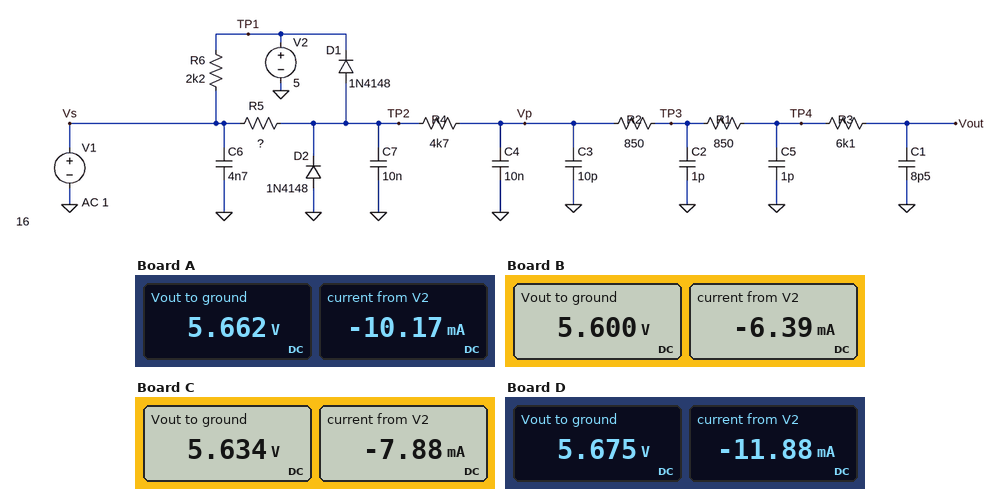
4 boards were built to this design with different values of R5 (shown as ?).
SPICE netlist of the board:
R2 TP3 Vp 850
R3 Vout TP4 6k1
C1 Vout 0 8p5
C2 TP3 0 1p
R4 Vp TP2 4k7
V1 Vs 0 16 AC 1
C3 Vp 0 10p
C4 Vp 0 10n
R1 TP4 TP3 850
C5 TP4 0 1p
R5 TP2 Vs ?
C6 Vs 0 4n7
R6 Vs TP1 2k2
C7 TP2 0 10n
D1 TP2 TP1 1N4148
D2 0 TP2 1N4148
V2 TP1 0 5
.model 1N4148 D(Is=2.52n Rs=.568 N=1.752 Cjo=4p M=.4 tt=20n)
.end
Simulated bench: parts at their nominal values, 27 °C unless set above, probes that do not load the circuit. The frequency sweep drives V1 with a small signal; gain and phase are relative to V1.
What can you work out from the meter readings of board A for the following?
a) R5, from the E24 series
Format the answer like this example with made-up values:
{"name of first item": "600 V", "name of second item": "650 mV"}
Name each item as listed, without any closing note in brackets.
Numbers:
{"R5, from the E24 series": "2 kΩ"}
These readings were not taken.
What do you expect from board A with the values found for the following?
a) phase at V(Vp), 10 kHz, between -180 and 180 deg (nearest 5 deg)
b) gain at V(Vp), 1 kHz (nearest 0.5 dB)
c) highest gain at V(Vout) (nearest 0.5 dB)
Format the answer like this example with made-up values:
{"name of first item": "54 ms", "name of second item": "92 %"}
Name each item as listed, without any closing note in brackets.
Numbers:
{"phase at V(Vp), 10 kHz, between -180 and 180 deg": "-70 deg", "gain at V(Vp), 1 kHz": "-47.0 dB", "highest gain at V(Vout)": "-46.5 dB"}
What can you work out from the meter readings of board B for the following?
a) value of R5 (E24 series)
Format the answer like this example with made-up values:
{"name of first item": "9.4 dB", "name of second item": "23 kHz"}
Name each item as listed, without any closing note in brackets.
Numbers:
{"value of R5": "7.5 kΩ"}
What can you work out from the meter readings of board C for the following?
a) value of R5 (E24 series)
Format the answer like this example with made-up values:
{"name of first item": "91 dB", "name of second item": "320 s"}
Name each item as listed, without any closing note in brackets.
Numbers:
{"value of R5": "3.6 kΩ"}
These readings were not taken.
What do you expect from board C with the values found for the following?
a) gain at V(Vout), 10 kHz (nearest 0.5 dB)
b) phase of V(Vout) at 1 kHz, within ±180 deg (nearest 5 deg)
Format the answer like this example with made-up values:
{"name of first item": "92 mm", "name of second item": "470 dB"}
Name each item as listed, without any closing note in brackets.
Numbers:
{"gain at V(Vout), 10 kHz": "-57.0 dB", "phase of V(Vout) at 1 kHz, within ±180 deg": "-15 deg"}
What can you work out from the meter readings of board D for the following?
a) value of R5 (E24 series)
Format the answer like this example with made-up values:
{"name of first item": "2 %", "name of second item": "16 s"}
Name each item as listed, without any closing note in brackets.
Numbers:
{"value of R5": "1.5 kΩ"}
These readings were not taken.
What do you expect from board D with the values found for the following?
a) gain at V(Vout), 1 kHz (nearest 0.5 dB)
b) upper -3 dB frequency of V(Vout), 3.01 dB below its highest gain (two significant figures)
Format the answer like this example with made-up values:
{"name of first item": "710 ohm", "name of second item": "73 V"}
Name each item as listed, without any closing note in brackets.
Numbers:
{"gain at V(Vout), 1 kHz": "-47.0 dB", "upper -3 dB frequency of V(Vout), 3.01 dB below its highest gain": "3.4 kHz"}
